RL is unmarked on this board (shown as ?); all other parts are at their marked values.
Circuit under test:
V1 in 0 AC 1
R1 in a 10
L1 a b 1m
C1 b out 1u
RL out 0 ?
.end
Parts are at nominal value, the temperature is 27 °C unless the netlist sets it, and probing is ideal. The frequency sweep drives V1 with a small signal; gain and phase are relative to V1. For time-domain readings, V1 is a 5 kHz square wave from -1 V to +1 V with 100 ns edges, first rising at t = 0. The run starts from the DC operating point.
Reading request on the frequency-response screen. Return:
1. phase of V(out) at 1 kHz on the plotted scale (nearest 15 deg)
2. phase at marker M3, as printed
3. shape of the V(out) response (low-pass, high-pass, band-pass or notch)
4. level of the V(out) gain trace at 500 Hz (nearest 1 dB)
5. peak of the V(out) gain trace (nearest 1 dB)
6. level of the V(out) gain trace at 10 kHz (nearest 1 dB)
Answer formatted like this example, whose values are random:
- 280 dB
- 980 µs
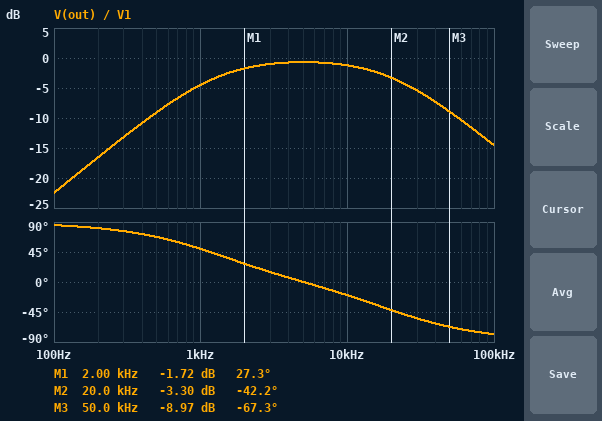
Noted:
- 45 deg
- -67.3 deg
- band-pass
- -9 dB
- -1 dB
- -1 dB
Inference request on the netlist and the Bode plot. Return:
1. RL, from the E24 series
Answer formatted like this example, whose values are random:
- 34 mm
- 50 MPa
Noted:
- 120 Ω
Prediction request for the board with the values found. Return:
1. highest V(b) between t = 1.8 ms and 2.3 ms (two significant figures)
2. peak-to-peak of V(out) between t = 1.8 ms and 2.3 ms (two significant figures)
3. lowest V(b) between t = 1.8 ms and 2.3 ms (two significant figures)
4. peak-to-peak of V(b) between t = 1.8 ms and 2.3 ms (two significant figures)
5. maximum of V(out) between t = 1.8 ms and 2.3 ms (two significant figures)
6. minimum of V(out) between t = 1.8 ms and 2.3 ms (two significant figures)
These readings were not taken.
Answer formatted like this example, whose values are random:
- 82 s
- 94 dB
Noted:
- 990 mV
- 2.2 V
- -990 mV
- 2.0 V
- 1.1 V
- -1.1 V
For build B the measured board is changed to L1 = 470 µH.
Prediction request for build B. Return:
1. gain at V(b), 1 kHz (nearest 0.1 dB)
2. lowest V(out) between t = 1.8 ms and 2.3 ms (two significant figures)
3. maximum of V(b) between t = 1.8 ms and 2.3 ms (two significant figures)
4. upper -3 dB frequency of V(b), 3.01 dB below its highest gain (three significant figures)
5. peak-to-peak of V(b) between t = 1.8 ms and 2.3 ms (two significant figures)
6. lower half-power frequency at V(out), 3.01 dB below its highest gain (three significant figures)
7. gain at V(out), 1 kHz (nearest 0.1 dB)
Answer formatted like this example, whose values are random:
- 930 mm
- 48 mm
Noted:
- -0.2 dB
- -1.2 V
- 970 mV
- 38.4 kHz
- 1.9 V
- 1.19 kHz
- -4.6 dB
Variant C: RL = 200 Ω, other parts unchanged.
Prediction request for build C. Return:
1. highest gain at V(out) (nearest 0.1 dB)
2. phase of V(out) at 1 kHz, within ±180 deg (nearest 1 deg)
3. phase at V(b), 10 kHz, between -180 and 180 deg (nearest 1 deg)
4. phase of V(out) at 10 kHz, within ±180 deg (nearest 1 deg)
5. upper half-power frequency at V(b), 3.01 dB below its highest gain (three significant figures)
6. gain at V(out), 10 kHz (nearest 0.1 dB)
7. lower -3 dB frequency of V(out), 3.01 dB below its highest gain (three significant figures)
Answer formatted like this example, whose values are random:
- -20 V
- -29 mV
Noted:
- -0.4 dB
- 36 deg
- -17 deg
- -13 deg
- 31.0 kHz
- -0.6 dB
- 741 Hz
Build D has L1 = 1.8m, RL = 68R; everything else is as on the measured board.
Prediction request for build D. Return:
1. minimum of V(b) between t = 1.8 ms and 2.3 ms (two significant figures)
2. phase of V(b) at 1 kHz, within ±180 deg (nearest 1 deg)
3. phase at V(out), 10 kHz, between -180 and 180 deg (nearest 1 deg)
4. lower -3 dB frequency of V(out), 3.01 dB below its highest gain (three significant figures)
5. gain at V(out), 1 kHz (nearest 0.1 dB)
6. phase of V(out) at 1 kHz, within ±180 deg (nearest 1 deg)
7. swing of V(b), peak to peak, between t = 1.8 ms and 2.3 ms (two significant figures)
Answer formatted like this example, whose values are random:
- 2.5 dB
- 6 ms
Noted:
- -1.1 V
- -5 deg
- -51 deg
- 1.65 kHz
- -7.8 dB
- 62 deg
- 2.3 V
